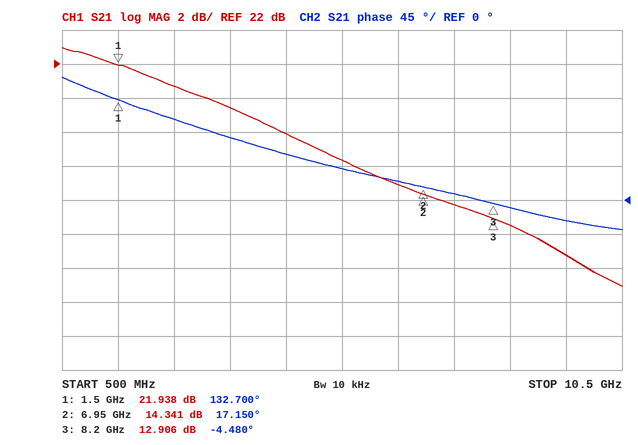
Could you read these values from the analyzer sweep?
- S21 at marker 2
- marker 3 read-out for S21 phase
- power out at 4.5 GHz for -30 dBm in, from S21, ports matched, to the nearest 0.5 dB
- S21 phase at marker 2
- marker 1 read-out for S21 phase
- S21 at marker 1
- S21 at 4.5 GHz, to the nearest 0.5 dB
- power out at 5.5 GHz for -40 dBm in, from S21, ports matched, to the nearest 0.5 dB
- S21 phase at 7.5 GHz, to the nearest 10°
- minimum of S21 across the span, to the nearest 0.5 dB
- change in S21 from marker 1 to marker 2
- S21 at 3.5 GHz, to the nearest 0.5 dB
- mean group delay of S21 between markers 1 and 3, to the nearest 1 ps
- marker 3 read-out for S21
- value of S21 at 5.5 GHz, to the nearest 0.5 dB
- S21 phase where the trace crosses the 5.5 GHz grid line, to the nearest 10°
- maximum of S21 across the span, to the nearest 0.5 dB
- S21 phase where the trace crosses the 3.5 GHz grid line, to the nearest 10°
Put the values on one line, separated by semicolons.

14.341 dB; -4.480°; -12.0 dBm; 17.150°; 132.700°; 21.938 dB; 18.0 dB; -23.5 dBm; 10°; 9.0 dB; -7.597 dB; 19.5 dB; 57 ps; 12.906 dB; 16.5 dB; 40°; 23.0 dB; 80°
